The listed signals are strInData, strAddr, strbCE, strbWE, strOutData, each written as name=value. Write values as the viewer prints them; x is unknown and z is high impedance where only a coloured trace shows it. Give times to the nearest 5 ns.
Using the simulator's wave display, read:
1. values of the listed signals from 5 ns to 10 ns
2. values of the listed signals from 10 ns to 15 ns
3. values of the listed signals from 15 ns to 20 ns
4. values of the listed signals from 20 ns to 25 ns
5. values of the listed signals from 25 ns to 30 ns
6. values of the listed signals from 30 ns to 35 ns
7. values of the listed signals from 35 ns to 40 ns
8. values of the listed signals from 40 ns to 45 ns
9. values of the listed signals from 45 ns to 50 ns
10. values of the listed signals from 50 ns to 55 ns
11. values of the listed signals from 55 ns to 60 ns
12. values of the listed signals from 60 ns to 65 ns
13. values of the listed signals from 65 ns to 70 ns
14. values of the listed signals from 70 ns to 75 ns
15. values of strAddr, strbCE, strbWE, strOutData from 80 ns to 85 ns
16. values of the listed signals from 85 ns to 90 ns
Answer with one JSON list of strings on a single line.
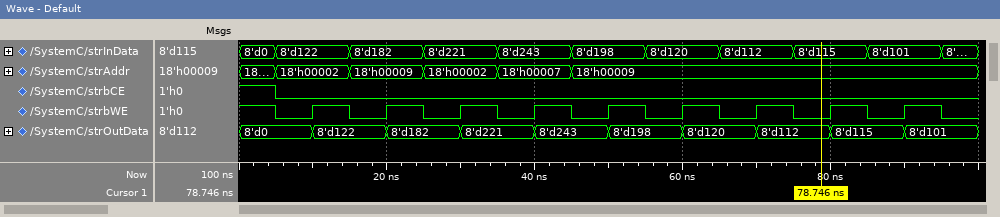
["strInData=8'd122, strAddr=18'h00002, strbCE=0, strbWE=0, strOutData=8'd0", "strInData=8'd122, strAddr=18'h00002, strbCE=0, strbWE=1, strOutData=8'd122", "strInData=8'd182, strAddr=18'h00009, strbCE=0, strbWE=0, strOutData=8'd122", "strInData=8'd182, strAddr=18'h00009, strbCE=0, strbWE=1, strOutData=8'd182", "strInData=8'd221, strAddr=18'h00002, strbCE=0, strbWE=0, strOutData=8'd182", "strInData=8'd221, strAddr=18'h00002, strbCE=0, strbWE=1, strOutData=8'd221", "strInData=8'd243, strAddr=18'h00007, strbCE=0, strbWE=0, strOutData=8'd221", "strInData=8'd243, strAddr=18'h00007, strbCE=0, strbWE=1, strOutData=8'd243", "strInData=8'd198, strAddr=18'h00009, strbCE=0, strbWE=0, strOutData=8'd243", "strInData=8'd198, strAddr=18'h00009, strbCE=0, strbWE=1, strOutData=8'd198", "strInData=8'd120, strAddr=18'h00009, strbCE=0, strbWE=0, strOutData=8'd198", "strInData=8'd120, strAddr=18'h00009, strbCE=0, strbWE=1, strOutData=8'd120", "strInData=8'd112, strAddr=18'h00009, strbCE=0, strbWE=0, strOutData=8'd120", "strInData=8'd112, strAddr=18'h00009, strbCE=0, strbWE=1, strOutData=8'd112", "strAddr=18'h00009, strbCE=0, strbWE=1, strOutData=8'd115", "strInData=8'd101, strAddr=18'h00009, strbCE=0, strbWE=0, strOutData=8'd115"]
